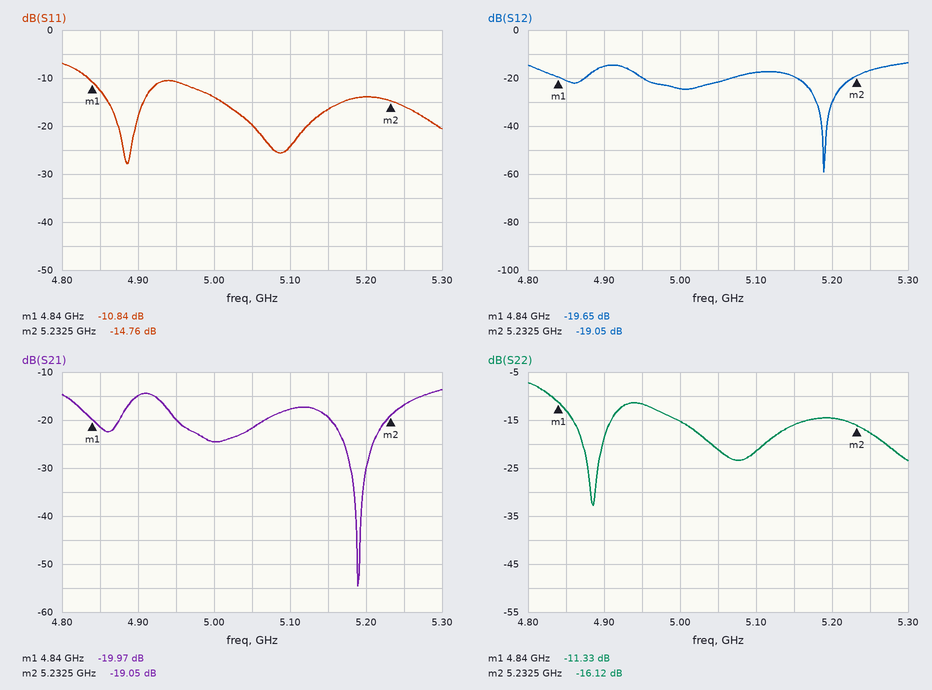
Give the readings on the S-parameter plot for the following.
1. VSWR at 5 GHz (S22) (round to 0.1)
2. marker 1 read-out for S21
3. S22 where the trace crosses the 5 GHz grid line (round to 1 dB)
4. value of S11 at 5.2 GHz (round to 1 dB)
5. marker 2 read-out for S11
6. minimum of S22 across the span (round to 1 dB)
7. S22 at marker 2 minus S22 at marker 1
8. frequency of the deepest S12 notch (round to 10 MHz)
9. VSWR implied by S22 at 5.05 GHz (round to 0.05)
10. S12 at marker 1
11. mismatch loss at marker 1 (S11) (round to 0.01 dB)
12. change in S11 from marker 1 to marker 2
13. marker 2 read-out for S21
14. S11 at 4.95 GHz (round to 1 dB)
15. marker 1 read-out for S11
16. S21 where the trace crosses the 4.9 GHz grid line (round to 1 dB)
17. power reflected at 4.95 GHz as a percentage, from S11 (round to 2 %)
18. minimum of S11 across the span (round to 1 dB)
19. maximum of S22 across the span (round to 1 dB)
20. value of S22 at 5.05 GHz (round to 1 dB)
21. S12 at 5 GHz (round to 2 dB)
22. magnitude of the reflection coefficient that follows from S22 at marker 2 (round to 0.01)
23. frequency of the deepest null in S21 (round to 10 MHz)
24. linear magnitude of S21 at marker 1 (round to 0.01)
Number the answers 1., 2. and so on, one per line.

1. 1.4
2. -19.97 dB
3. -15 dB
4. -14 dB
5. -14.76 dB
6. -33 dB
7. -4.79 dB
8. 5.19 GHz
9. 1.20
10. -19.65 dB
11. 0.37 dB
12. -3.92 dB
13. -19.05 dB
14. -11 dB
15. -10.84 dB
16. -15 dB
17. 8 %
18. -28 dB
19. -7 dB
20. -21 dB
21. -24 dB
22. 0.16
23. 5.19 GHz
24. 0.10
